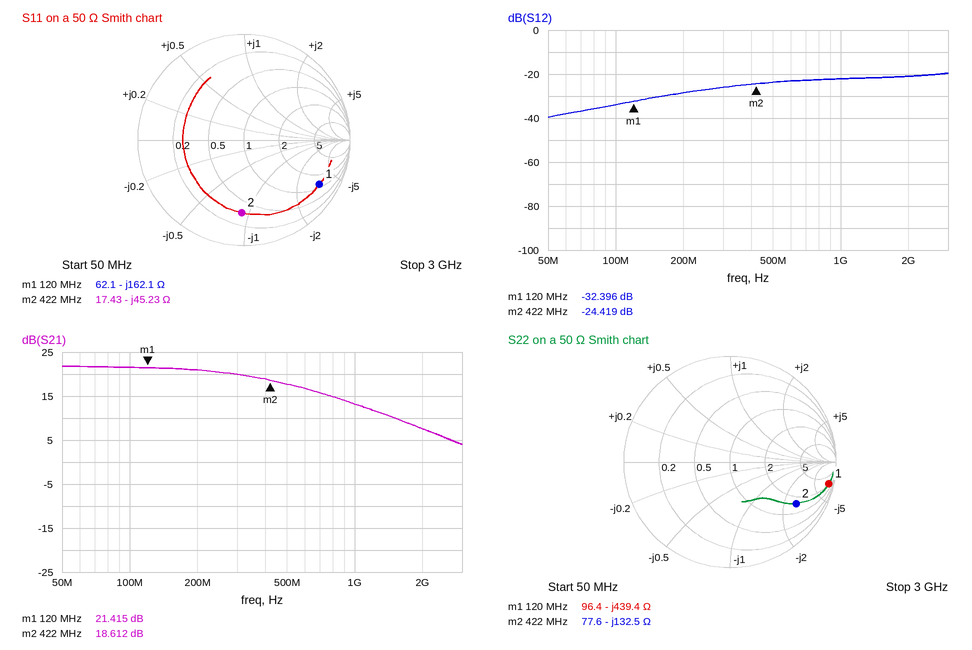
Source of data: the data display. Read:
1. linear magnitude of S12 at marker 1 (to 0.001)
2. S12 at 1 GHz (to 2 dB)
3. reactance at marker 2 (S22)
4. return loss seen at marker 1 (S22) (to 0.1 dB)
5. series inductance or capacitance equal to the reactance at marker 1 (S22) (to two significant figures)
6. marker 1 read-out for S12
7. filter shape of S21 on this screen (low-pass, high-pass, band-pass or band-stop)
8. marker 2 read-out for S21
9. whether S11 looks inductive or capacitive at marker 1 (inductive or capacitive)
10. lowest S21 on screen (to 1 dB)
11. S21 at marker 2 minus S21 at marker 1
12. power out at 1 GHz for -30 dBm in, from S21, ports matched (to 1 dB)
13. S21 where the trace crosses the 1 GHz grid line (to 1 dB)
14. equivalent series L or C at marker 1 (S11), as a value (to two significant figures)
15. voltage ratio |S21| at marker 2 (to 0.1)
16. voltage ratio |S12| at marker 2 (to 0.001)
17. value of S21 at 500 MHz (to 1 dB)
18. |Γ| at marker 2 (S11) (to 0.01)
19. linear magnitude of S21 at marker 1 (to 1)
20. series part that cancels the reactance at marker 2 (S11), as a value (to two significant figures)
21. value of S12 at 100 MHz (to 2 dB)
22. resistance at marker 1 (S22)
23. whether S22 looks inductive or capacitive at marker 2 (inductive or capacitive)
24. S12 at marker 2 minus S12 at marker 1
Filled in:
0.024
-22 dB
-132.5 Ω
0.4 dB
3.0 pF
-32.396 dB
low-pass
18.612 dB
capacitive
4 dB
-2.803 dB
-17 dBm
13 dB
8.2 pF
8.5
0.060
18 dB
0.69
12
17 nH
-34 dB
96.4 Ω
capacitive
7.977 dB
